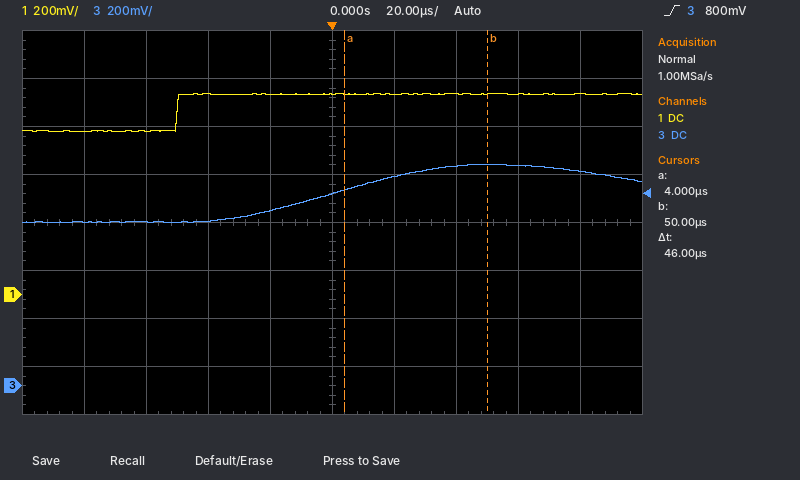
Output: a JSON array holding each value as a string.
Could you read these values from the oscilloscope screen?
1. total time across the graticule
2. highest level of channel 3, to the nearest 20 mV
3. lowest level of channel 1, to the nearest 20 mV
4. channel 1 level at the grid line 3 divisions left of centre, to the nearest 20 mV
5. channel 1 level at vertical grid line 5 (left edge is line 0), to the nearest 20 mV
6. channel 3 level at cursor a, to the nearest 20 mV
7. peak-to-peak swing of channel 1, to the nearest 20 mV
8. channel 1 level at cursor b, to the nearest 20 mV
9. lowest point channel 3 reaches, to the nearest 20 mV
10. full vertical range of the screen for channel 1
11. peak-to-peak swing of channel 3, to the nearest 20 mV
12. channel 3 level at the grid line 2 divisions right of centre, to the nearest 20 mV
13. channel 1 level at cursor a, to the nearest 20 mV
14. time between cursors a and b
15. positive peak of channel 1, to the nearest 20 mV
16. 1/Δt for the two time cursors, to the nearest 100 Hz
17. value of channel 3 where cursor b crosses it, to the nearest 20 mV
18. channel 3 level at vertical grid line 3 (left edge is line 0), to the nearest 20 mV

["200 µs", "920 mV", "680 mV", "680 mV", "840 mV", "820 mV", "160 mV", "840 mV", "680 mV", "1.6 V", "240 mV", "920 mV", "840 mV", "46 µs", "840 mV", "21.7 kHz", "920 mV", "680 mV"]
